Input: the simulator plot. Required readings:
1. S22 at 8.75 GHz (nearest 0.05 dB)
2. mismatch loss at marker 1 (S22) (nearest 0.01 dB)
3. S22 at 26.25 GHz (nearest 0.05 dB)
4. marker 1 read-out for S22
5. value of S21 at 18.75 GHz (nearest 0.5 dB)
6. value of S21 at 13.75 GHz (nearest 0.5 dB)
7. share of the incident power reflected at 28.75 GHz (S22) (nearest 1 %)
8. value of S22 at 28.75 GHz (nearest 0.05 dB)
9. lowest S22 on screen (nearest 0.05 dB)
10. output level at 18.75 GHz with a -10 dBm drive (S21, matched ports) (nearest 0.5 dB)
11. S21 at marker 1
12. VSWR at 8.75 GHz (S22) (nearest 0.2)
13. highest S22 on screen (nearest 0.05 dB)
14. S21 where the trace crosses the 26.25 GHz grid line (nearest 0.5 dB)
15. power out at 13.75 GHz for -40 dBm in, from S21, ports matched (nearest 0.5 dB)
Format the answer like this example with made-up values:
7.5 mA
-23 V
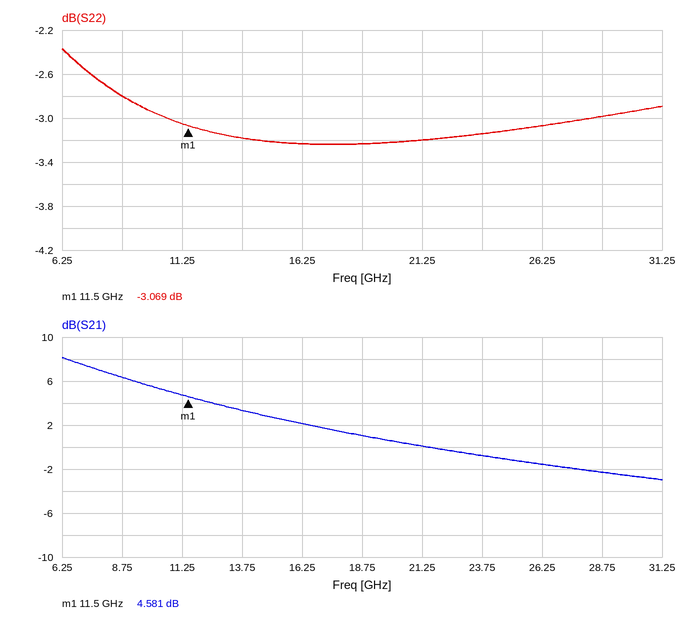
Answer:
-2.80 dB
2.95 dB
-3.05 dB
-3.069 dB
1.0 dB
3.5 dB
50 %
-3.00 dB
-3.25 dB
-9.0 dBm
4.581 dB
6.2
-2.35 dB
-1.5 dB
-36.5 dBm
